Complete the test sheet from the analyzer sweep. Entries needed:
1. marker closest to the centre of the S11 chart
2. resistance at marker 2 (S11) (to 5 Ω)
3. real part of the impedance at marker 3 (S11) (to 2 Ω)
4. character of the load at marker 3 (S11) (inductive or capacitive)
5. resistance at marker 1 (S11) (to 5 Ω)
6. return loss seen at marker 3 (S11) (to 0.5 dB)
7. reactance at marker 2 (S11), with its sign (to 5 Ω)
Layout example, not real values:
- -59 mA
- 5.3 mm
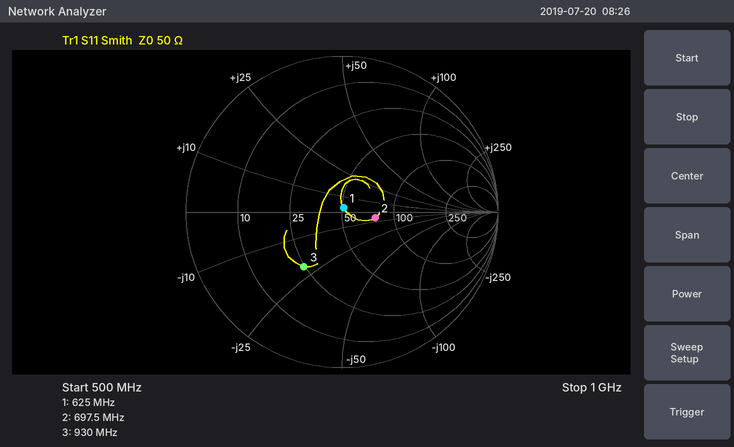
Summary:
- marker 1
- 75 Ω
- 24 Ω
- capacitive
- 50 Ω
- 7.5 dB
- -5 Ω
